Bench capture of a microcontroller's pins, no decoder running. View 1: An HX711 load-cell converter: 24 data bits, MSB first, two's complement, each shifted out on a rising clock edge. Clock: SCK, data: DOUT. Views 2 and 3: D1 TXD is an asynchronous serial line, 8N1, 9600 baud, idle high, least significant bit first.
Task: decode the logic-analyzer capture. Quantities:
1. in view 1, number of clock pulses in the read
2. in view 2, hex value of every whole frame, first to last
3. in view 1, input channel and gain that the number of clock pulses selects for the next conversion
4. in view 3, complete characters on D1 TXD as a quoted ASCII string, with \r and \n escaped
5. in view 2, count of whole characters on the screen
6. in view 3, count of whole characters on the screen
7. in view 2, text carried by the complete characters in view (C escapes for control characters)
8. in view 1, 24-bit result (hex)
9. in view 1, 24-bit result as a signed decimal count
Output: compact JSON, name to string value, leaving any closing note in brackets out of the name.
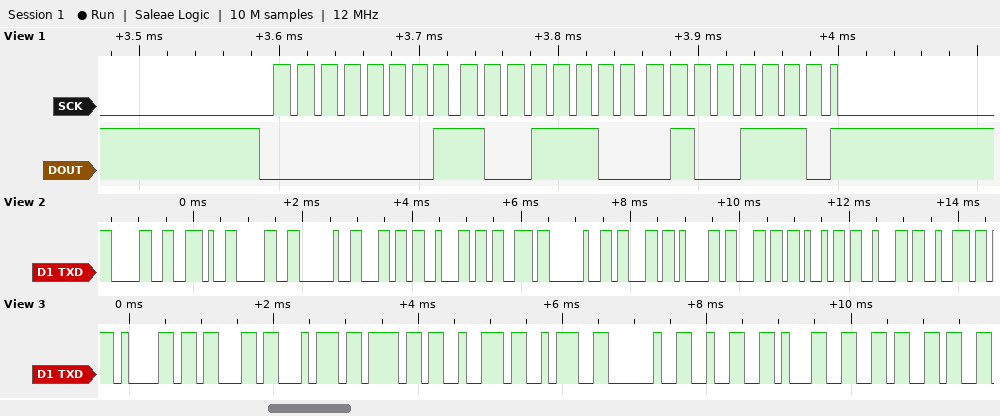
{"in view 1, number of clock pulses in the read": "25", "in view 2, hex value of every whole frame, first to last": "0x30 0x2E 0x30 0x20 0x6C 0x62 0x73 0x20 0x63 0x61 0x6C 0x69 0x62 0x72", "in view 1, input channel and gain that the number of clock pulses selects for the next conversion": "channel A, gain 128", "in view 3, complete characters on D1 TXD as a quoted ASCII string, with \\r and \\n escaped": "\"actor: 216\"", "in view 2, count of whole characters on the screen": "14", "in view 3, count of whole characters on the screen": "10", "in view 2, text carried by the complete characters in view": "\"0.0 lbs calibr\"", "in view 1, 24-bit result": "0x019C4E", "in view 1, 24-bit result as a signed decimal count": "105550"}
